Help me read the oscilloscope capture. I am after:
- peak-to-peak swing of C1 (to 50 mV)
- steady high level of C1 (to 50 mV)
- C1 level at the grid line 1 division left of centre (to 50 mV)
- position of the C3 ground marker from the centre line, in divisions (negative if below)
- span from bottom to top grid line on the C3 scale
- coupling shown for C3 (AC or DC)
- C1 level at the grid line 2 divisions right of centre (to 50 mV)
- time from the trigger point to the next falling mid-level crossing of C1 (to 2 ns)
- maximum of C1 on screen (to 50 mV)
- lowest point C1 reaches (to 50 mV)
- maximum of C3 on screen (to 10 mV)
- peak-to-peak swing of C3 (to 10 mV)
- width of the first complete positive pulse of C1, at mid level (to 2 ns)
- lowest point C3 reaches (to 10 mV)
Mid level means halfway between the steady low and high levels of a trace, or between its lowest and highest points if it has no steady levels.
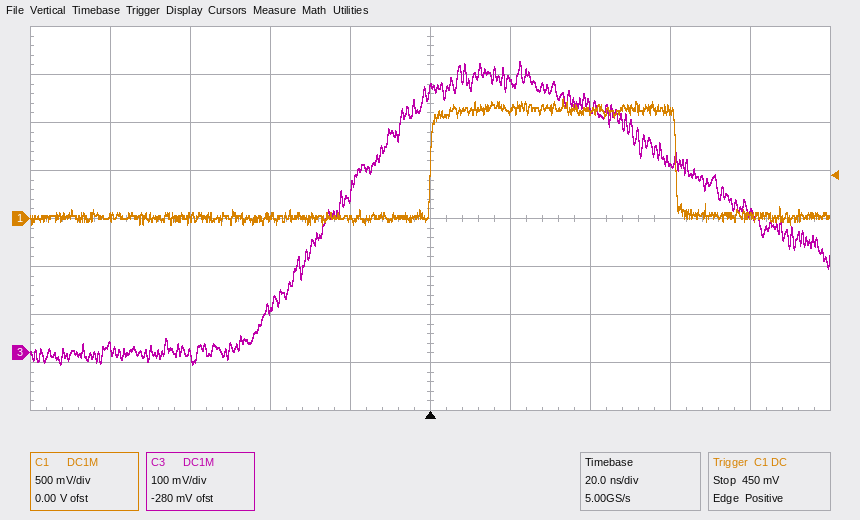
1.30 V
1.15 V
0 mV
-2.8 div
800 mV
DC
1.10 V
62 ns
1.25 V
-50 mV
610 mV
630 mV
62 ns
-20 mV
